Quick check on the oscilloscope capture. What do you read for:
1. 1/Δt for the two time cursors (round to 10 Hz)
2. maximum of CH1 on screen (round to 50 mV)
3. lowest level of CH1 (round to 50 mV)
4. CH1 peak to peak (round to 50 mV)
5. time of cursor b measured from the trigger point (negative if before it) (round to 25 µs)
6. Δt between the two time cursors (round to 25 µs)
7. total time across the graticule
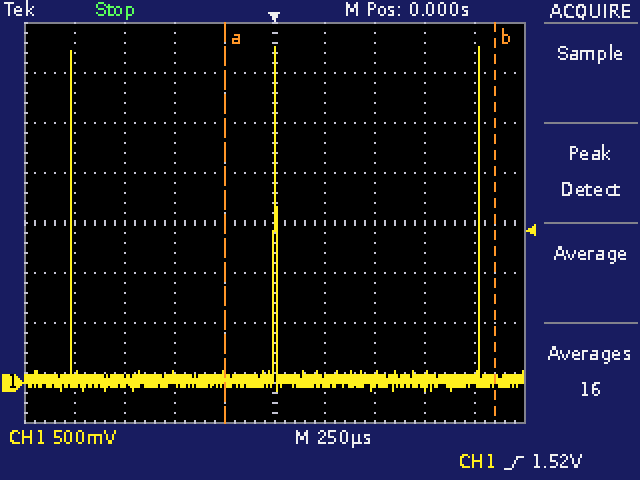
740 Hz
3.35 V
-100 mV
3.45 V
+1.100 ms
1.350 ms
2.5 ms
